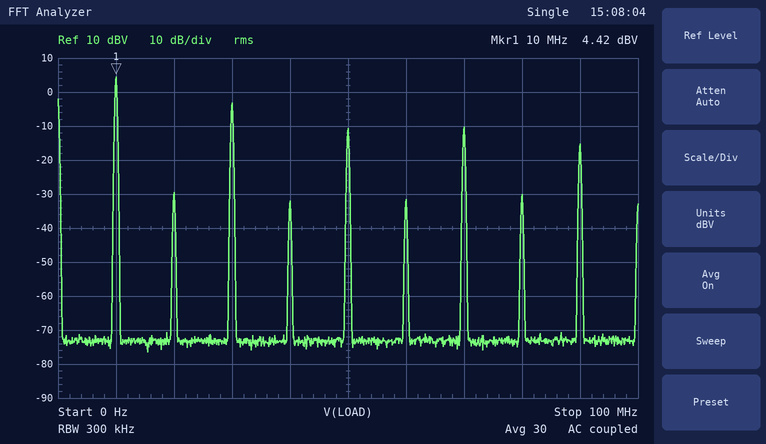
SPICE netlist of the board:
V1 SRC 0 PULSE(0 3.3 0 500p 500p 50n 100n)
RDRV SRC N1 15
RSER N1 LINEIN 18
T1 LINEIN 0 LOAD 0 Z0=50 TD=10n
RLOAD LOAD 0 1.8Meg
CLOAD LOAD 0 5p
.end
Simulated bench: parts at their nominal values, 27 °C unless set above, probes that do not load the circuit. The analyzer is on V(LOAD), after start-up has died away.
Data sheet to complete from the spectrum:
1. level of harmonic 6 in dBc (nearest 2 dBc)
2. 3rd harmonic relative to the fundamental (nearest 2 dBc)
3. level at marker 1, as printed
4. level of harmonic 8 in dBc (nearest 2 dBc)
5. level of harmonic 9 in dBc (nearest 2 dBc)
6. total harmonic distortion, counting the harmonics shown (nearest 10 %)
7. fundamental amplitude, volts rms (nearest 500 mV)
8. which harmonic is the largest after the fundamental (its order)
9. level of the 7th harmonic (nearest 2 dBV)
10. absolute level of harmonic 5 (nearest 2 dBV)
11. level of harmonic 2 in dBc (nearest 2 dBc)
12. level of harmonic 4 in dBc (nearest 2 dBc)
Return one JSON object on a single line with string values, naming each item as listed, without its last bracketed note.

{"level of harmonic 6 in dBc": "-36 dBc", "3rd harmonic relative to the fundamental": "-8 dBc", "level at marker 1, as printed": "4.42 dBV", "level of harmonic 8 in dBc": "-34 dBc", "level of harmonic 9 in dBc": "-20 dBc", "total harmonic distortion, counting the harmonics shown": "50 %", "fundamental amplitude, volts rms": "1.5 V", "which harmonic is the largest after the fundamental": "3", "level of the 7th harmonic": "-10 dBV", "absolute level of harmonic 5": "-10 dBV", "level of harmonic 2 in dBc": "-34 dBc", "level of harmonic 4 in dBc": "-36 dBc"}
